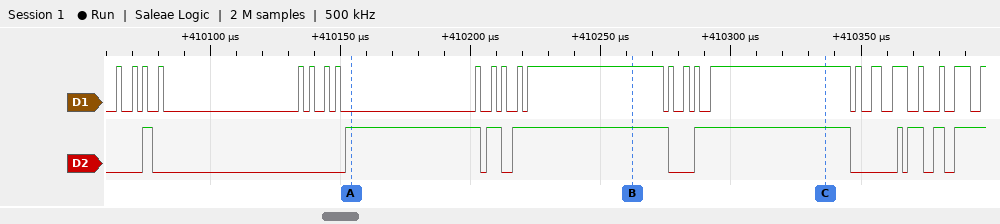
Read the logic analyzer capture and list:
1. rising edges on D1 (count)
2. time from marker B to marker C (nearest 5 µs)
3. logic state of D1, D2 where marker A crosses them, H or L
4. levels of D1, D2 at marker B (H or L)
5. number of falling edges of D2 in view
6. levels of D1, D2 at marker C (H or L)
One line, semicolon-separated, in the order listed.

24; 75 µs; D1=L, D2=H; D1=H, D2=H; 8; D1=H, D2=H
